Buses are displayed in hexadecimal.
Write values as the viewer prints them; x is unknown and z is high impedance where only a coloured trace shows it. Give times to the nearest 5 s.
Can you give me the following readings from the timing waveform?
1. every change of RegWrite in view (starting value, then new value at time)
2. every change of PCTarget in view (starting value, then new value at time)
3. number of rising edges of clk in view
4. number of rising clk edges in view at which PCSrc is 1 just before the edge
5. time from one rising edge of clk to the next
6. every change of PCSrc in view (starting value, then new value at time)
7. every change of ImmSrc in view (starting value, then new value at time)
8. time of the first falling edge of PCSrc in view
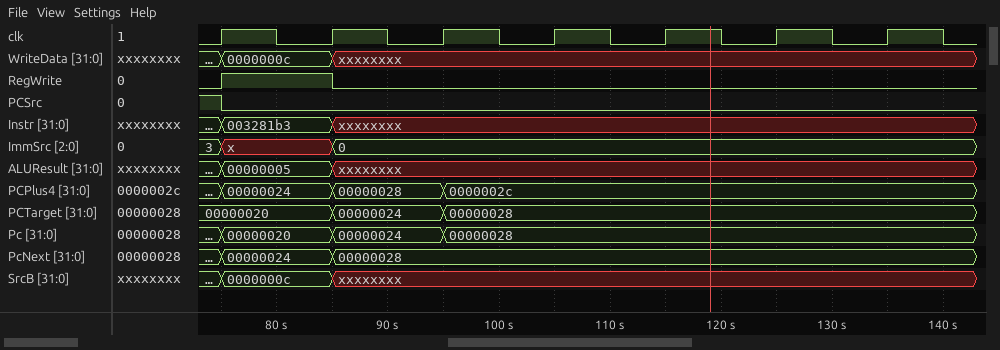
0, 1 at 75 s, 0 at 85 s
00000020, 00000024 at 85 s, 00000028 at 95 s
7
1
10 s
1, 0 at 75 s
3, x at 75 s, 0 at 85 s
75 s
